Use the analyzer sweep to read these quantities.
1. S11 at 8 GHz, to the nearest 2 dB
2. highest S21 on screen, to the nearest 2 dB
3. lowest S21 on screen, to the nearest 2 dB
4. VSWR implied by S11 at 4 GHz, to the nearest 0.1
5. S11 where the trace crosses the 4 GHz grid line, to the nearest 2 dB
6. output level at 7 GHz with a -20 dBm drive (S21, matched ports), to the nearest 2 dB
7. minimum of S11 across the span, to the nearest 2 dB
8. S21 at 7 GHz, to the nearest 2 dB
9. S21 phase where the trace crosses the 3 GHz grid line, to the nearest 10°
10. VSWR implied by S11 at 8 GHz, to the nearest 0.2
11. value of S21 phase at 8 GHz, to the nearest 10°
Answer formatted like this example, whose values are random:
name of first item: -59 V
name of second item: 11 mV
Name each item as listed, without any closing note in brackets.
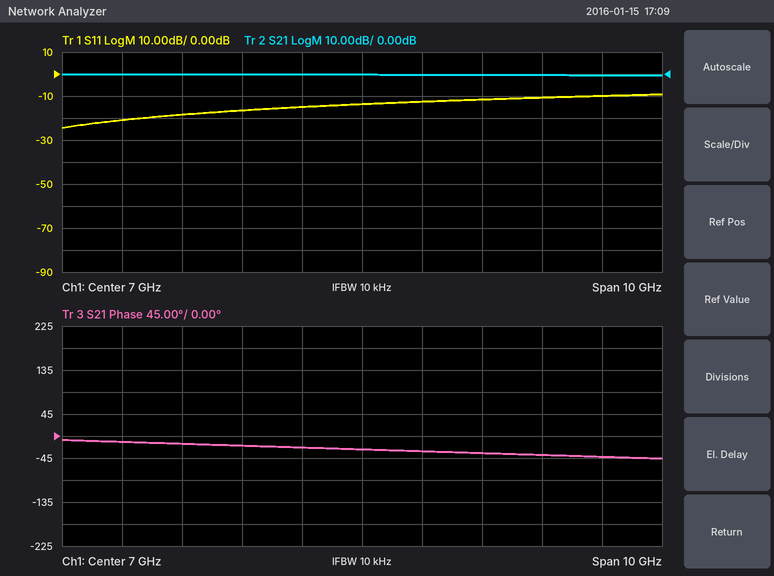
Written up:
S11 at 8 GHz, to the nearest 2 dB: -12 dB
highest S21 on screen, to the nearest 2 dB: 0 dB
lowest S21 on screen, to the nearest 2 dB: 0 dB
VSWR implied by S11 at 4 GHz, to the nearest 0.1: 1.3
S11 where the trace crosses the 4 GHz grid line, to the nearest 2 dB: -18 dB
output level at 7 GHz with a -20 dBm drive (S21, matched ports), to the nearest 2 dB: -20 dBm
minimum of S11 across the span, to the nearest 2 dB: -24 dB
S21 at 7 GHz, to the nearest 2 dB: 0 dB
S21 phase where the trace crosses the 3 GHz grid line, to the nearest 10°: -10°
VSWR implied by S11 at 8 GHz, to the nearest 0.2: 1.6
value of S21 phase at 8 GHz, to the nearest 10°: -30°
